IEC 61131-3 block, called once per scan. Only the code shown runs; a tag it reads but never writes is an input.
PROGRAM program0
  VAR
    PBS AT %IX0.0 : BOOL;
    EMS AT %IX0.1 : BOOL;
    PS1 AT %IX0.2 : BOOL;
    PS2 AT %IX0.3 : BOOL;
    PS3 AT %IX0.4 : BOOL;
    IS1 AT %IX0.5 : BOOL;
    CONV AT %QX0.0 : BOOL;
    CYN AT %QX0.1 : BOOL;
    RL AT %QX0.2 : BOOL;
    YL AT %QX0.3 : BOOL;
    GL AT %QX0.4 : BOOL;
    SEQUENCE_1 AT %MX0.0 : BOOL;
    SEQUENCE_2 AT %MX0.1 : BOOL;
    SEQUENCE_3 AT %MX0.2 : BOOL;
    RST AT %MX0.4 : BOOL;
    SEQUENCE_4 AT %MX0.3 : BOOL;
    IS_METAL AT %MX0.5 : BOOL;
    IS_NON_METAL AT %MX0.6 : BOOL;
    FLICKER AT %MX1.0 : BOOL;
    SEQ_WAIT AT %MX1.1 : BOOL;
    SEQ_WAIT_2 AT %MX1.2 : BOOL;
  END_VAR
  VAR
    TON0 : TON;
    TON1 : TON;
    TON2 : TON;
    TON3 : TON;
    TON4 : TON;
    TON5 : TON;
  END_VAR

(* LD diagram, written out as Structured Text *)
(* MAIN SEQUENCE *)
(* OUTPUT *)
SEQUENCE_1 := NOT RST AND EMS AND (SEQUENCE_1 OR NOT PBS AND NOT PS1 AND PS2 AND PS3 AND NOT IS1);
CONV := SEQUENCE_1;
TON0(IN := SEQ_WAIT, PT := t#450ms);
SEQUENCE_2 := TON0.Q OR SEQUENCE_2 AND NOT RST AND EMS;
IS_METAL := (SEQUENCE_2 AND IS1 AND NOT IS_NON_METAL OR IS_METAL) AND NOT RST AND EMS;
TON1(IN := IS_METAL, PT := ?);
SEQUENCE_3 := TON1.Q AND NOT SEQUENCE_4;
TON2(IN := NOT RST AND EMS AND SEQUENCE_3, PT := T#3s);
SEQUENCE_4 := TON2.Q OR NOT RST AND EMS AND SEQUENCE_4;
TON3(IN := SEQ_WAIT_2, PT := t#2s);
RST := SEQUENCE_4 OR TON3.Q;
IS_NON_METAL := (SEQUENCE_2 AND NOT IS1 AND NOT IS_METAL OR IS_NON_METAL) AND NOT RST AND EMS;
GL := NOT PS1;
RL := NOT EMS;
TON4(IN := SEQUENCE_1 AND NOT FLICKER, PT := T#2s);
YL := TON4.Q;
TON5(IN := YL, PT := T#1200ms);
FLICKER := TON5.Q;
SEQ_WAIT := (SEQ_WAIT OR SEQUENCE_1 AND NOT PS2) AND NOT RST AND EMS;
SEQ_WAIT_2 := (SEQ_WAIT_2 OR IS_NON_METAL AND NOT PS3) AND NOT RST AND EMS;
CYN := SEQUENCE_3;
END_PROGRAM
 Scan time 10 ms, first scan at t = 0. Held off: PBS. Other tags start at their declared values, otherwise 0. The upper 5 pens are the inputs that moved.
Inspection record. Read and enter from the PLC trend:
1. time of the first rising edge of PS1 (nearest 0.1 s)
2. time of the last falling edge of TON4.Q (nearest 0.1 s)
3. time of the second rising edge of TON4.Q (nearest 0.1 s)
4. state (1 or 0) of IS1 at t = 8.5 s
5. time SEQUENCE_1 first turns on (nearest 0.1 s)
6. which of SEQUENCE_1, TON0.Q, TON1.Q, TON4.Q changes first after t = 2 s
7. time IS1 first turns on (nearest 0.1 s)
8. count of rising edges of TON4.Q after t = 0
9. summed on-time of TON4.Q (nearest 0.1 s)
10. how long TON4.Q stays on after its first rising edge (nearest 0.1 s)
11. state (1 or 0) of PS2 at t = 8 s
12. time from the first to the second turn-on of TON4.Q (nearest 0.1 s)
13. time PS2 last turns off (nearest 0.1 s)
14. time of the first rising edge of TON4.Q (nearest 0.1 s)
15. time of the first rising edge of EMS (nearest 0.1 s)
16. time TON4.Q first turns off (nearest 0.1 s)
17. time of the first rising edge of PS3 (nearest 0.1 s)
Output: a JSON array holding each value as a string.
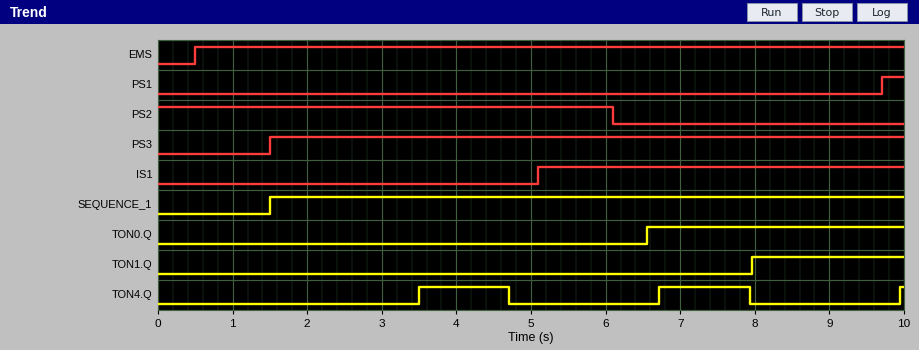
["9.7 s", "7.9 s", "6.7 s", "1", "1.5 s", "TON4.Q", "5.1 s", "3", "2.5 s", "1.2 s", "0", "3.2 s", "6.1 s", "3.5 s", "0.5 s", "4.7 s", "1.5 s"]
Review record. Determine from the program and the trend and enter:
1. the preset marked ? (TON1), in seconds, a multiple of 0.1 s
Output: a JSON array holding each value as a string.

["1.4 s"]
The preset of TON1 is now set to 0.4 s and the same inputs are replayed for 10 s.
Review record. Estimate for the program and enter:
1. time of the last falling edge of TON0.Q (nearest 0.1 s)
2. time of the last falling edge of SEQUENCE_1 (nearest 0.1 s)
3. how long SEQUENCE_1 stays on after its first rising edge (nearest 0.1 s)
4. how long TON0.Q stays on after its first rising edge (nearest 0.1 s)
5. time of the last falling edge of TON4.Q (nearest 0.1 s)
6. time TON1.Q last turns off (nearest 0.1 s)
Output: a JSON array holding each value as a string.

["10.0 s", "10.0 s", "8.5 s", "3.4 s", "10.0 s", "10.0 s"]
